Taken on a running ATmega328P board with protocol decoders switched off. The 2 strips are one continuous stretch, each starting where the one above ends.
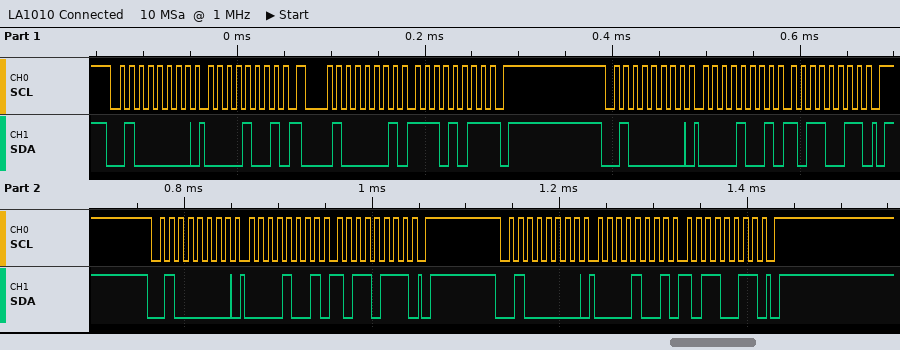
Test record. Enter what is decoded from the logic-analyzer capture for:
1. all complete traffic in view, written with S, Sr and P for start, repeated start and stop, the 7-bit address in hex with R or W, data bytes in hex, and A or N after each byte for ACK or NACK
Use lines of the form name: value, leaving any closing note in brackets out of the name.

all complete traffic in view, written with S, Sr and P for start, repeated start and stop, the 7-bit address in hex with R or W, data bytes in hex, and A or N after each byte for ACK or NACK: S 20W A 09 A Sr 20R A EB N P S 20W A 09 A B3 A P S 20W A 09 A B7 A P S 20W A 09 A B3 A P
